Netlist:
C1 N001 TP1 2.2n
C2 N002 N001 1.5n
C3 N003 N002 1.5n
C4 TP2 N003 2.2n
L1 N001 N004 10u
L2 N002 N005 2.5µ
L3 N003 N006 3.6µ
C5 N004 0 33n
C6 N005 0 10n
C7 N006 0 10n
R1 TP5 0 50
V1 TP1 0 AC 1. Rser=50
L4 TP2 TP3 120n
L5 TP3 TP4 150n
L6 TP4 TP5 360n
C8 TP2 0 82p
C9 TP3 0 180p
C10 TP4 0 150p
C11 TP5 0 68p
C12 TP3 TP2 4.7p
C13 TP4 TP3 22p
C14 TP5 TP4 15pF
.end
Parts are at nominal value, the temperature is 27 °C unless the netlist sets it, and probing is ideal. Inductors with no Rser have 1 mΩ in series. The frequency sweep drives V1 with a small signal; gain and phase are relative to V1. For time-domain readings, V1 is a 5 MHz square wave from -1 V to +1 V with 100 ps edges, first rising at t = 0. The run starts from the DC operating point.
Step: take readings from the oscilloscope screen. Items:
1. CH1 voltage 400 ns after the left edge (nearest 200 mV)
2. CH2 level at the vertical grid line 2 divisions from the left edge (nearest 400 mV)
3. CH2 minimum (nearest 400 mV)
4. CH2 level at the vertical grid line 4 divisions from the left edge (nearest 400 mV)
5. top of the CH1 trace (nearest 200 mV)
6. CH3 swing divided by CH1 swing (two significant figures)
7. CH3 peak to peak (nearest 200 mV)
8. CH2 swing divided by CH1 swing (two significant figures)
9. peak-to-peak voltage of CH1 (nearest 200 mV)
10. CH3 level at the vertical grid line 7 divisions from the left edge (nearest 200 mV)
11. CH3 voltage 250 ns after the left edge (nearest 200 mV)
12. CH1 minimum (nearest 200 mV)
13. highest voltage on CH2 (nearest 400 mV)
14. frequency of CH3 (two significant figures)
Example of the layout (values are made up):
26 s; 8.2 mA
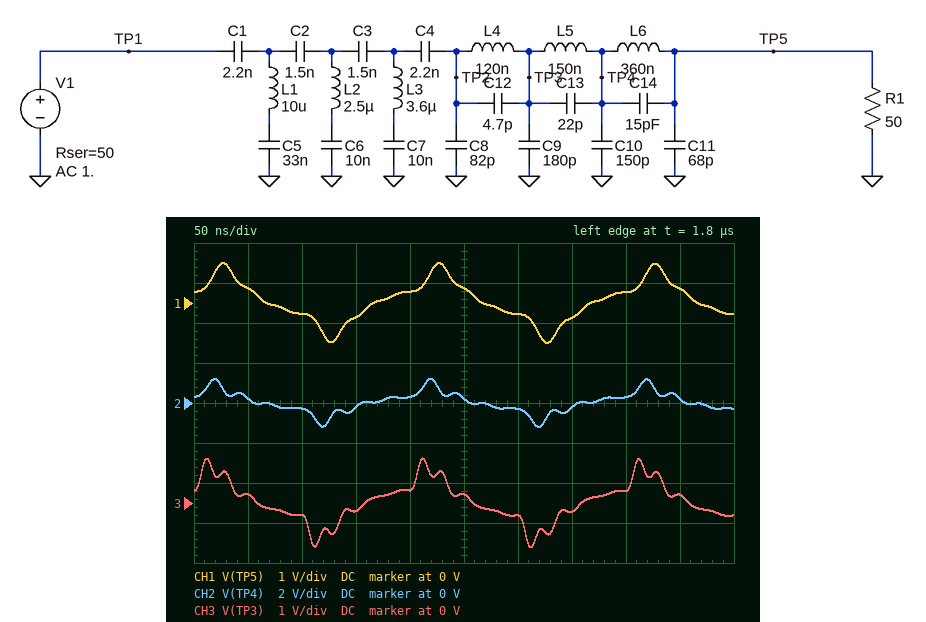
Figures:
200 mV; -400 mV; -1.2 V; 400 mV; 1.0 V; 1.1; 2.2 V; 1.2; 2.0 V; -200 mV; 200 mV; -1.0 V; 1.2 V; 5.0 MHz
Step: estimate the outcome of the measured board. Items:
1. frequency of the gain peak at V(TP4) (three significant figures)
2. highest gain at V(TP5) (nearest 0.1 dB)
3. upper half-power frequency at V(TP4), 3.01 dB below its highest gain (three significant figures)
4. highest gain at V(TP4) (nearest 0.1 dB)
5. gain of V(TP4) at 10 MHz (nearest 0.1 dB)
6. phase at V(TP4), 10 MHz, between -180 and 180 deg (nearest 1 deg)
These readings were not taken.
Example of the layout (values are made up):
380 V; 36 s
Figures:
39.3 MHz; -6.0 dB; 43.6 MHz; 0.8 dB; -6.4 dB; 0 deg
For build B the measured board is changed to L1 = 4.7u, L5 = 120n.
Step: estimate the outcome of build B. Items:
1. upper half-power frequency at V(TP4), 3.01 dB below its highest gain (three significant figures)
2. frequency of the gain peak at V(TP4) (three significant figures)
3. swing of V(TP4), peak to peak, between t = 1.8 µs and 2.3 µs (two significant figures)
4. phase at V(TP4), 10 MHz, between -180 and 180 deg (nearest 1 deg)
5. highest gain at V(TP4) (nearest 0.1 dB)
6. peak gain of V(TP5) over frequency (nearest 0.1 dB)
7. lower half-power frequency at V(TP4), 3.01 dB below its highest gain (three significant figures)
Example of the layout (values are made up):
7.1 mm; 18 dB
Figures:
49.1 MHz; 42.7 MHz; 2.5 V; 4 deg; 0 dB; -6.1 dB; 35.9 MHz
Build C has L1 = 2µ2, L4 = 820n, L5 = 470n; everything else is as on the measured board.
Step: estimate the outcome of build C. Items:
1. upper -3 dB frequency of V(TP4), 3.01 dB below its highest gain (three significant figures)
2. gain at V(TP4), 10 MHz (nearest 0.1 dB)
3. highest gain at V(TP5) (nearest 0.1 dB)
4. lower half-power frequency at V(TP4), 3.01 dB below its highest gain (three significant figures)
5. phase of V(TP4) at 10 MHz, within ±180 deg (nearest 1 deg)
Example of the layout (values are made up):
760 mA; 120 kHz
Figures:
27.0 MHz; -6.5 dB; -6.1 dB; 1.66 MHz; -31 deg
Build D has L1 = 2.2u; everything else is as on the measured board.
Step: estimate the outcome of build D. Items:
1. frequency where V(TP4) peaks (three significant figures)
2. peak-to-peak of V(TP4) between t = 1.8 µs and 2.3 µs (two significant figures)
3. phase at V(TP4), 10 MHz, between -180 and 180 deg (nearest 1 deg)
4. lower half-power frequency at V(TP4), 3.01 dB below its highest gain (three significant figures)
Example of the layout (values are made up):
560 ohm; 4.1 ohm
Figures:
39.6 MHz; 2.3 V; 9 deg; 34.4 MHz
